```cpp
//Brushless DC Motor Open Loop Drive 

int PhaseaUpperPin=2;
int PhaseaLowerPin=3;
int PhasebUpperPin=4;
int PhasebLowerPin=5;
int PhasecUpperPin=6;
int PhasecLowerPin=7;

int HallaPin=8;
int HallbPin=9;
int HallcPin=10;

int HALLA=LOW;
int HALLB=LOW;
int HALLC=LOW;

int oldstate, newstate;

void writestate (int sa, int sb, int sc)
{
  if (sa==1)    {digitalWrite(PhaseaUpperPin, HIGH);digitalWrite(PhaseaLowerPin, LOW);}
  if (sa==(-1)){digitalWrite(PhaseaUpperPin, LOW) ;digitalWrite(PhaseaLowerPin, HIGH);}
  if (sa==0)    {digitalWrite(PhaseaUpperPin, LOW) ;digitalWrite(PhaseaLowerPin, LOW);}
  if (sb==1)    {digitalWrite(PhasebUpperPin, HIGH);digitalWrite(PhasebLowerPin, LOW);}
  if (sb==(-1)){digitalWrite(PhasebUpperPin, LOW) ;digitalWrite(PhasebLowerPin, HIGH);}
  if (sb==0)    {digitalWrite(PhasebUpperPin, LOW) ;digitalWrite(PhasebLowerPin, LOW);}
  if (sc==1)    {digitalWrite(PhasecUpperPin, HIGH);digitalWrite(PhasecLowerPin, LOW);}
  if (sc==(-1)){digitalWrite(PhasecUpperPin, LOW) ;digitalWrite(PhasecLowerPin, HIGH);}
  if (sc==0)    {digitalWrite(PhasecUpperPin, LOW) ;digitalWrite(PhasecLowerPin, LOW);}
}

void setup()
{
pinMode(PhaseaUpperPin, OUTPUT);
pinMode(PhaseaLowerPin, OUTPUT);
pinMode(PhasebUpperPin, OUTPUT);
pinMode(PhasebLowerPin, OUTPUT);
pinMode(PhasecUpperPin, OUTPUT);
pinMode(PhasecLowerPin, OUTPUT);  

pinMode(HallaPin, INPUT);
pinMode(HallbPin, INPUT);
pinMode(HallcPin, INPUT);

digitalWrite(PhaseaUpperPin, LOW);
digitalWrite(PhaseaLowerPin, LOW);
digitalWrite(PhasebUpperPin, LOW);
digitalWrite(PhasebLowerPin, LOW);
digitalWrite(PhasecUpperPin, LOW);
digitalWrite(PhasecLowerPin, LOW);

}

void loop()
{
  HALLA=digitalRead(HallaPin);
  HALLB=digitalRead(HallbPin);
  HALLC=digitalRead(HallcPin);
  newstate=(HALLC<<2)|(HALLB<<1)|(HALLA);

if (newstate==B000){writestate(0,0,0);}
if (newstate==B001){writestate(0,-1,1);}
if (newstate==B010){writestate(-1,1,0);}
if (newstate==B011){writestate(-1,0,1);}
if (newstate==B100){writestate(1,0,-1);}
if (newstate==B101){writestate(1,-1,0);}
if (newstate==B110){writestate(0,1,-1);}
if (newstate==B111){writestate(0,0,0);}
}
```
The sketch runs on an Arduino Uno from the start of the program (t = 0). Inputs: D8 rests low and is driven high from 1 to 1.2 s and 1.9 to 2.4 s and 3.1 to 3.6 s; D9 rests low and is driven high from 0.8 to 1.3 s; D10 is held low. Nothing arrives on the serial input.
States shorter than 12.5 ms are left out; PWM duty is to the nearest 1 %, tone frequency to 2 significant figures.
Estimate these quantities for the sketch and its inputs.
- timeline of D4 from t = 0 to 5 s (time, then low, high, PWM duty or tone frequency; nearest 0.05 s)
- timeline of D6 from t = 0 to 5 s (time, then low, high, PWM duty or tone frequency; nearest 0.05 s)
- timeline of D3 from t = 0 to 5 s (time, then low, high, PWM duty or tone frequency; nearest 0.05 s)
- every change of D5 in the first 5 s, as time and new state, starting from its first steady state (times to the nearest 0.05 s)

0 s low; 0.8 s high; 1 s low; 1.2 s high; 1.3 s low
0 s low; 1 s high; 1.2 s low; 1.9 s high; 2.4 s low; 3.1 s high; 3.6 s low
0 s low; 0.8 s high; 1.3 s low
0 s low; 1.9 s high; 2.4 s low; 3.1 s high; 3.6 s low
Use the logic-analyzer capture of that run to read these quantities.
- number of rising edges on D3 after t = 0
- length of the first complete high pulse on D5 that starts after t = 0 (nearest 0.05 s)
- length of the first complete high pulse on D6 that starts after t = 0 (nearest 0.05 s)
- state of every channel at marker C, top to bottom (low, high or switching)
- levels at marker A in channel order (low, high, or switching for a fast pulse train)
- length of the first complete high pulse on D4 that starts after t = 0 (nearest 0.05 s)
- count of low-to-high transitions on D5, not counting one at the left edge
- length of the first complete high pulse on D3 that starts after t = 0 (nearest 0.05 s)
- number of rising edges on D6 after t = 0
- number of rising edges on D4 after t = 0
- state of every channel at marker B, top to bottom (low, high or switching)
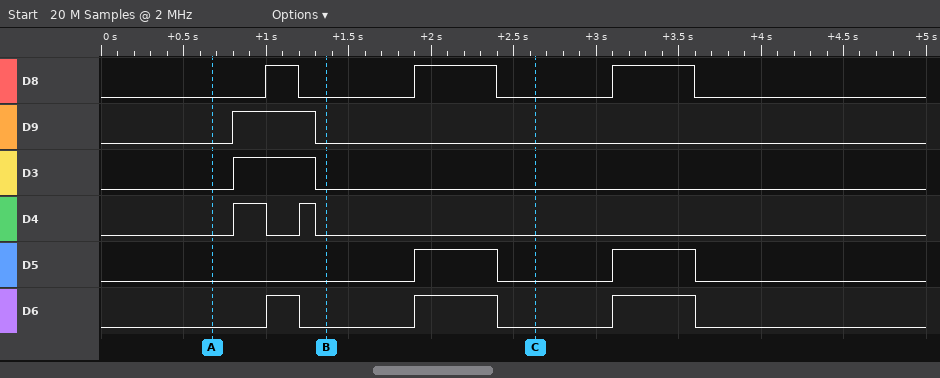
1
0.50 s
0.20 s
D8 low, D9 low, D3 low, D4 low, D5 low, D6 low
D8 low, D9 low, D3 low, D4 low, D5 low, D6 low
0.20 s
2
0.50 s
3
2
D8 low, D9 low, D3 low, D4 low, D5 low, D6 low
